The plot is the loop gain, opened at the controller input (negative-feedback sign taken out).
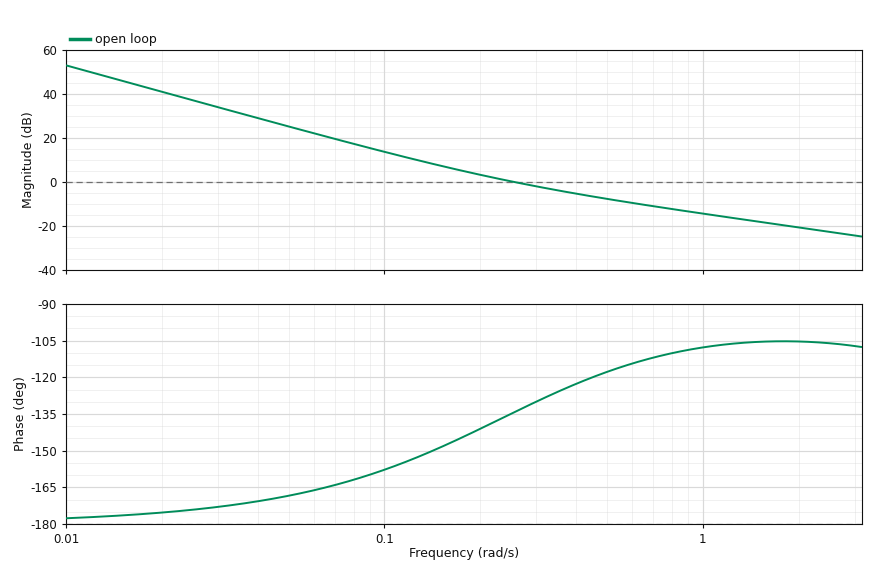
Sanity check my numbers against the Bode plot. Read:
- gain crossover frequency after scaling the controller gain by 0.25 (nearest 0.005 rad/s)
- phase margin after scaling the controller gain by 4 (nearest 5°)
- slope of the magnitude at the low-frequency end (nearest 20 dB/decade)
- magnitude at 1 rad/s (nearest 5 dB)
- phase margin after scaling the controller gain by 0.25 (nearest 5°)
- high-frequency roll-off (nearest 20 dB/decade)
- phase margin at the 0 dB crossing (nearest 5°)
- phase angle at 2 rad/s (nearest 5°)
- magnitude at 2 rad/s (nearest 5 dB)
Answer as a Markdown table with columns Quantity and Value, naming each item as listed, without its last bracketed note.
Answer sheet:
| Quantity | Value |
|---|---|
| gain crossover frequency after scaling the controller gain by 0.25 | 0.110 rad/s |
| phase margin after scaling the controller gain by 4 | 70° |
| slope of the magnitude at the low-frequency end | -40 dB/decade |
| magnitude at 1 rad/s | -15 dB |
| phase margin after scaling the controller gain by 0.25 | 25° |
| high-frequency roll-off | -20 dB/decade |
| phase margin at the 0 dB crossing | 45° |
| phase angle at 2 rad/s | -105° |
| magnitude at 2 rad/s | -20 dB |
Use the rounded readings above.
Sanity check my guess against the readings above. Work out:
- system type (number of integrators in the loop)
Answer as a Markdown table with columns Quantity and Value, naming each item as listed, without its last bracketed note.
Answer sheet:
| Quantity | Value |
|---|---|
| system type | 2 |
